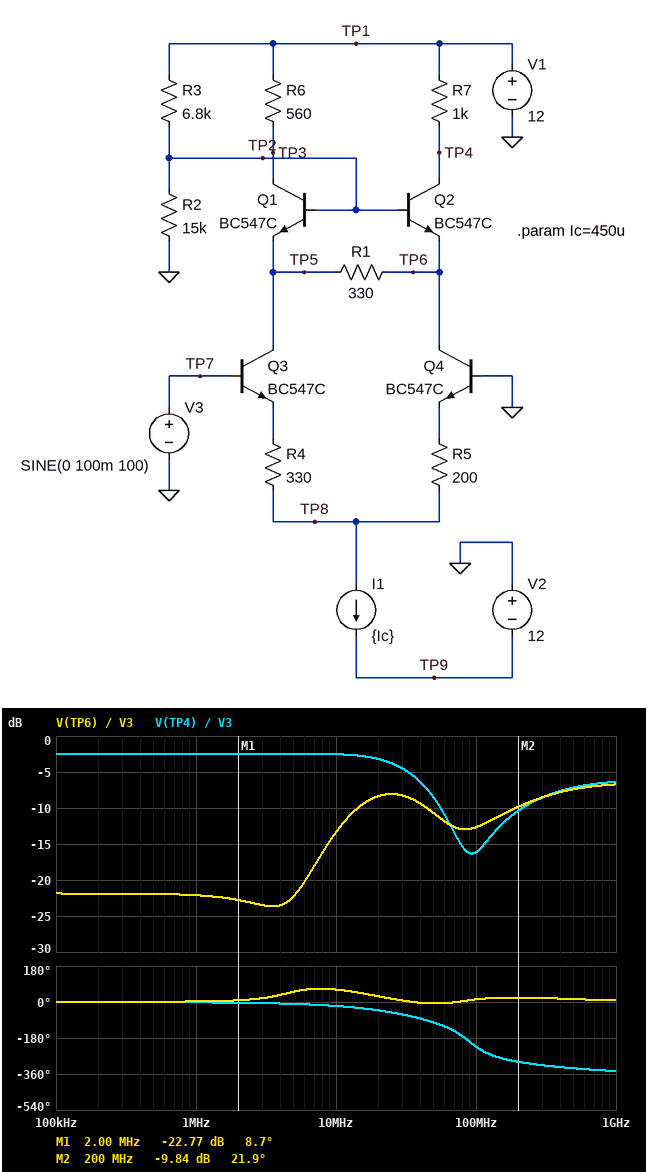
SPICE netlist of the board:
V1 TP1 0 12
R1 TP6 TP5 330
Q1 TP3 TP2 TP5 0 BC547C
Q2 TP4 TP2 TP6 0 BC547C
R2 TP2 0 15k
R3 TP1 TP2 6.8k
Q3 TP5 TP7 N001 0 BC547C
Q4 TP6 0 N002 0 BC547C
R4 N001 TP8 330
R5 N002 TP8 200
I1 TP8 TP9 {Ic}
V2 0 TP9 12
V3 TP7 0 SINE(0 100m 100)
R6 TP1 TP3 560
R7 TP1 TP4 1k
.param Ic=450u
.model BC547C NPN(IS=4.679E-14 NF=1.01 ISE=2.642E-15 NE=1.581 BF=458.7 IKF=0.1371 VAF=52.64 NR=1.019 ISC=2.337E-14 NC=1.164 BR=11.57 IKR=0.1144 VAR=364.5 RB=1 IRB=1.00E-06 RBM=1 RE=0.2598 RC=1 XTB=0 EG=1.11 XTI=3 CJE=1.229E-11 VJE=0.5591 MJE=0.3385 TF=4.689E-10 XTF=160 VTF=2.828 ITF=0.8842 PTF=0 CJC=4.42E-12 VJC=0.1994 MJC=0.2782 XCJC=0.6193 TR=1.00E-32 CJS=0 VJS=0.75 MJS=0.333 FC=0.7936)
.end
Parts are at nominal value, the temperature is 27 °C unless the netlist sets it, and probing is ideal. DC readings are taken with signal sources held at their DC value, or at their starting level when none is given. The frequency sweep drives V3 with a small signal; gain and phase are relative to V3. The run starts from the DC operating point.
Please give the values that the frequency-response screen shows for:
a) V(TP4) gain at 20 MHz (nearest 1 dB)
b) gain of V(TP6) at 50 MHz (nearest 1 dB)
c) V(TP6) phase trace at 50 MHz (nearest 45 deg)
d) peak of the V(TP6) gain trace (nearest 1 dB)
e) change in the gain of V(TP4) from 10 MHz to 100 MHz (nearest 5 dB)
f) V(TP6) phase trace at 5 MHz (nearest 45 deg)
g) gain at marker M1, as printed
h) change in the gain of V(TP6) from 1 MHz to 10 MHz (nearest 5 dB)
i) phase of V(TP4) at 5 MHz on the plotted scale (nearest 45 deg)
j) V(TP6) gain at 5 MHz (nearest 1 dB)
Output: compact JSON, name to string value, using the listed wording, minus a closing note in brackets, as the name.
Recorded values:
{"V(TP4) gain at 20 MHz": "-3 dB", "gain of V(TP6) at 50 MHz": "-11 dB", "V(TP6) phase trace at 50 MHz": "0 deg", "peak of the V(TP6) gain trace": "-7 dB", "change in the gain of V(TP4) from 10 MHz to 100 MHz": "-15 dB", "V(TP6) phase trace at 5 MHz": "45 deg", "gain at marker M1, as printed": "-22.77 dB", "change in the gain of V(TP6) from 1 MHz to 10 MHz": "10 dB", "phase of V(TP4) at 5 MHz on the plotted scale": "0 deg", "V(TP6) gain at 5 MHz": "-22 dB"}
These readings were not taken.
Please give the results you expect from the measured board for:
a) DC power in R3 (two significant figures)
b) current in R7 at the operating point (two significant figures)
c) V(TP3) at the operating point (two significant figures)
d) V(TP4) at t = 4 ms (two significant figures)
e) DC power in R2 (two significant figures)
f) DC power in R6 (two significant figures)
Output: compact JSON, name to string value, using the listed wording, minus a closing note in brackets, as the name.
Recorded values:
{"DC power in R3": "2.1 mW", "current in R7 at the operating point": "250 µA", "V(TP3) at the operating point": "12 V", "V(TP4) at t = 4 ms": "12 V", "DC power in R2": "4.5 mW", "DC power in R6": "23 µW"}
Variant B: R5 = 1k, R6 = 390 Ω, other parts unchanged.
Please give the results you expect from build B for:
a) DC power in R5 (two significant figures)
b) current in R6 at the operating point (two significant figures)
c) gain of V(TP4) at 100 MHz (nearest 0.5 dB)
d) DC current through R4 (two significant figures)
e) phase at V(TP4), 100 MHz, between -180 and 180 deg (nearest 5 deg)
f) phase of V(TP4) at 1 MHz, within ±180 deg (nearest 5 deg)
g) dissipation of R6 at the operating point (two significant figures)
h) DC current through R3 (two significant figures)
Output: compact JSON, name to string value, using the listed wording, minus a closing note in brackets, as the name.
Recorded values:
{"DC power in R5": "17 µW", "current in R6 at the operating point": "280 µA", "gain of V(TP4) at 100 MHz": "-13.5 dB", "DC current through R4": "320 µA", "phase at V(TP4), 100 MHz, between -180 and 180 deg": "100 deg", "phase of V(TP4) at 1 MHz, within ±180 deg": "-5 deg", "dissipation of R6 at the operating point": "30 µW", "DC current through R3": "550 µA"}
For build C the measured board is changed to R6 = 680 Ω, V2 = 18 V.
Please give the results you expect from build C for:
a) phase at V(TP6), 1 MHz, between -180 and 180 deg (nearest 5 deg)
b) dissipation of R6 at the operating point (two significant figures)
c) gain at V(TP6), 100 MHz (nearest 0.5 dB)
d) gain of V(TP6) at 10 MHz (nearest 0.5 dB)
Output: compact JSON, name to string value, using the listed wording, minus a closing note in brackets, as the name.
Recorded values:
{"phase at V(TP6), 1 MHz, between -180 and 180 deg": "0 deg", "dissipation of R6 at the operating point": "28 µW", "gain at V(TP6), 100 MHz": "-12.0 dB", "gain of V(TP6) at 10 MHz": "-14.0 dB"}
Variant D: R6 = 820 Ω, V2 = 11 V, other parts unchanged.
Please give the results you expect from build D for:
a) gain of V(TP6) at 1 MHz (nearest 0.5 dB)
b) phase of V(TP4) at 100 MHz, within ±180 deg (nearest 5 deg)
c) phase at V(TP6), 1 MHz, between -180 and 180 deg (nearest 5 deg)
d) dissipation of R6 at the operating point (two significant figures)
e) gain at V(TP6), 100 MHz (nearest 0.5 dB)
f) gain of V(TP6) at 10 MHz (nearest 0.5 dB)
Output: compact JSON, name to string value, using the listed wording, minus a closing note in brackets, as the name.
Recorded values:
{"gain of V(TP6) at 1 MHz": "-22.5 dB", "phase of V(TP4) at 100 MHz, within ±180 deg": "130 deg", "phase at V(TP6), 1 MHz, between -180 and 180 deg": "-5 deg", "dissipation of R6 at the operating point": "33 µW", "gain at V(TP6), 100 MHz": "-11.5 dB", "gain of V(TP6) at 10 MHz": "-14.0 dB"}
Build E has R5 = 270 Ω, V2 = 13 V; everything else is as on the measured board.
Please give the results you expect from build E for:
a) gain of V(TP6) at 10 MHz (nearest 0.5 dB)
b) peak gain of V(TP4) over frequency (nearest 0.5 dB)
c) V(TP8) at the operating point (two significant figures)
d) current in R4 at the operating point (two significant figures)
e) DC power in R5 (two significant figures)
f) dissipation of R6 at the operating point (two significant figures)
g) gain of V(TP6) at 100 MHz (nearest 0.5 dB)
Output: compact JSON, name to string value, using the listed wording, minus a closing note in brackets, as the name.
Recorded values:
{"gain of V(TP6) at 10 MHz": "-15.0 dB", "peak gain of V(TP4) over frequency": "-3.0 dB", "V(TP8) at the operating point": "-650 mV", "current in R4 at the operating point": "210 µA", "DC power in R5": "16 µW", "dissipation of R6 at the operating point": "26 µW", "gain of V(TP6) at 100 MHz": "-12.0 dB"}
